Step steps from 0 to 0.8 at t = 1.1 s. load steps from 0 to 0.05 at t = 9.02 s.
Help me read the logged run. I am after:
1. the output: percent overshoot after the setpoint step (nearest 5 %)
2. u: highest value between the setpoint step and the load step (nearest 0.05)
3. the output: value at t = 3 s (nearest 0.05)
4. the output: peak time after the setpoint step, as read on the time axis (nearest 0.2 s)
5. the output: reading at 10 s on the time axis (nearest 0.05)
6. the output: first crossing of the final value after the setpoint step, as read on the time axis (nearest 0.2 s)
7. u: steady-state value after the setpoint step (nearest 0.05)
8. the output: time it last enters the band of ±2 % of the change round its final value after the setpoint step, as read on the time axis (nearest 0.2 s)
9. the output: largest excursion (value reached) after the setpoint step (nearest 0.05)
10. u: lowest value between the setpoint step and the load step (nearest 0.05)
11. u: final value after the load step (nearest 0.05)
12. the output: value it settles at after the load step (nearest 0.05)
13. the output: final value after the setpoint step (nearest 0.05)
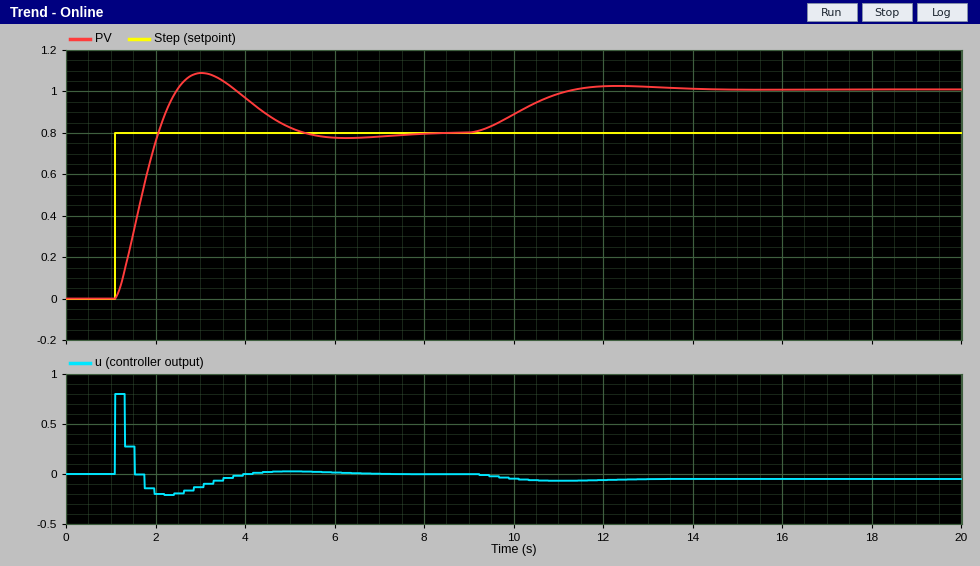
35 %
0.80
1.10
3.0 s
0.90
2.0 s
0.00
7.2 s
1.10
-0.20
-0.05
1.00
0.80
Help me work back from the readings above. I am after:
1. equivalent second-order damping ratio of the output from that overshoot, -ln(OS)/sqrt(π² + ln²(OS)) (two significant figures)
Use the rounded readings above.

0.32
